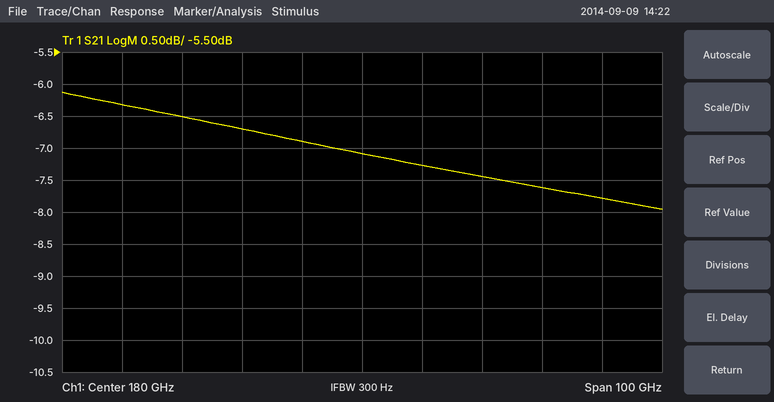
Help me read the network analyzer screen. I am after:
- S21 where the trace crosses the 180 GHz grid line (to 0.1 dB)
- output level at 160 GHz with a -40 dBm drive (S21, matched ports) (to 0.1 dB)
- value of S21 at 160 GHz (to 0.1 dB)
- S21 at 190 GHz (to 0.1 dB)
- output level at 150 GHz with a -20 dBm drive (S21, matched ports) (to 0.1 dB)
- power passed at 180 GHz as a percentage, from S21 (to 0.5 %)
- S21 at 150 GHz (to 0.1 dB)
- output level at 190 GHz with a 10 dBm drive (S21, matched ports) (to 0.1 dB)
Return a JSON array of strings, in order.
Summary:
["-7.1 dB", "-46.7 dBm", "-6.7 dB", "-7.3 dB", "-26.5 dBm", "19.5 %", "-6.5 dB", "2.7 dBm"]
